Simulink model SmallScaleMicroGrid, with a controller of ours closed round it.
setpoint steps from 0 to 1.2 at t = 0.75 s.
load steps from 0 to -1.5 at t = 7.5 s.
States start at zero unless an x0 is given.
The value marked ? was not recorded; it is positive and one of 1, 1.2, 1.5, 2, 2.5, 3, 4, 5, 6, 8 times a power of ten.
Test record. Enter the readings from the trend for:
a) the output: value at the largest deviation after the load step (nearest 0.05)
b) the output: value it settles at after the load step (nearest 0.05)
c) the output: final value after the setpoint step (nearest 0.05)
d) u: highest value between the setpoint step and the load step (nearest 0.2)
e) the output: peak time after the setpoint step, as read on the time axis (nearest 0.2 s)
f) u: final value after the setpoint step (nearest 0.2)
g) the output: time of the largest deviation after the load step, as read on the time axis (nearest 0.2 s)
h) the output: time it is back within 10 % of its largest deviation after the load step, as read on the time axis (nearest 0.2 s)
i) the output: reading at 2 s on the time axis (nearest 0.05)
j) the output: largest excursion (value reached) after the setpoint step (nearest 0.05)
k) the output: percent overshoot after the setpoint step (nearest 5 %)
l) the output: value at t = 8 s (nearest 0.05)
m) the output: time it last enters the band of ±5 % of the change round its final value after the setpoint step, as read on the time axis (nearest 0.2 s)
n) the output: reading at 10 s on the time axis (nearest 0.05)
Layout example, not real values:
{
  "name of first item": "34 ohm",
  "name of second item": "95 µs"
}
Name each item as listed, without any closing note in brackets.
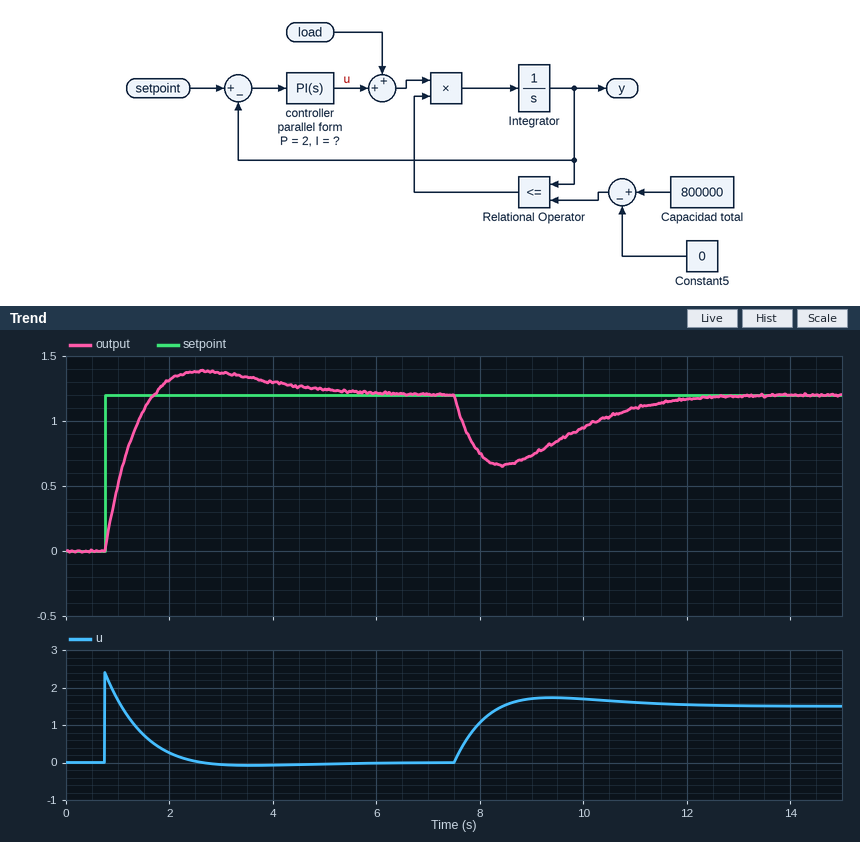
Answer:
{
  "the output: value at the largest deviation after the load step": "0.65",
  "the output: value it settles at after the load step": "1.20",
  "the output: final value after the setpoint step": "1.20",
  "u: highest value between the setpoint step and the load step": "2.4",
  "the output: peak time after the setpoint step, as read on the time axis": "2.6 s",
  "u: final value after the setpoint step": "0.0",
  "the output: time of the largest deviation after the load step, as read on the time axis": "8.4 s",
  "the output: time it is back within 10 % of its largest deviation after the load step, as read on the time axis": "11.6 s",
  "the output: reading at 2 s on the time axis": "1.30",
  "the output: largest excursion (value reached) after the setpoint step": "1.40",
  "the output: percent overshoot after the setpoint step": "15 %",
  "the output: value at t = 8 s": "0.75",
  "the output: time it last enters the band of ±5 % of the change round its final value after the setpoint step, as read on the time axis": "4.6 s",
  "the output: reading at 10 s on the time axis": "0.95"
}
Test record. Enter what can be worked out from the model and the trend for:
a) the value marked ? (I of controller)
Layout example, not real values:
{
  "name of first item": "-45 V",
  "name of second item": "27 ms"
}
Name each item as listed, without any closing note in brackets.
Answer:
{
  "the value marked ?": "1.2"
}
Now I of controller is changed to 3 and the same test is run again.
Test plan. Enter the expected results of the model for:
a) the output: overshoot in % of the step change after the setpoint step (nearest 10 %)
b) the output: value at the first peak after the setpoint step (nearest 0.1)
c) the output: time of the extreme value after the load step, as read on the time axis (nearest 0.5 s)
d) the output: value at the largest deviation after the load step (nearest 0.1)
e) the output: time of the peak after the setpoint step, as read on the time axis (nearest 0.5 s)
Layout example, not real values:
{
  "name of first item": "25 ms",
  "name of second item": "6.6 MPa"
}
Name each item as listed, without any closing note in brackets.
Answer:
{
  "the output: overshoot in % of the step change after the setpoint step": "30 %",
  "the output: value at the first peak after the setpoint step": "1.5",
  "the output: time of the extreme value after the load step, as read on the time axis": "8.0 s",
  "the output: value at the largest deviation after the load step": "0.8",
  "the output: time of the peak after the setpoint step, as read on the time axis": "2.0 s"
}
